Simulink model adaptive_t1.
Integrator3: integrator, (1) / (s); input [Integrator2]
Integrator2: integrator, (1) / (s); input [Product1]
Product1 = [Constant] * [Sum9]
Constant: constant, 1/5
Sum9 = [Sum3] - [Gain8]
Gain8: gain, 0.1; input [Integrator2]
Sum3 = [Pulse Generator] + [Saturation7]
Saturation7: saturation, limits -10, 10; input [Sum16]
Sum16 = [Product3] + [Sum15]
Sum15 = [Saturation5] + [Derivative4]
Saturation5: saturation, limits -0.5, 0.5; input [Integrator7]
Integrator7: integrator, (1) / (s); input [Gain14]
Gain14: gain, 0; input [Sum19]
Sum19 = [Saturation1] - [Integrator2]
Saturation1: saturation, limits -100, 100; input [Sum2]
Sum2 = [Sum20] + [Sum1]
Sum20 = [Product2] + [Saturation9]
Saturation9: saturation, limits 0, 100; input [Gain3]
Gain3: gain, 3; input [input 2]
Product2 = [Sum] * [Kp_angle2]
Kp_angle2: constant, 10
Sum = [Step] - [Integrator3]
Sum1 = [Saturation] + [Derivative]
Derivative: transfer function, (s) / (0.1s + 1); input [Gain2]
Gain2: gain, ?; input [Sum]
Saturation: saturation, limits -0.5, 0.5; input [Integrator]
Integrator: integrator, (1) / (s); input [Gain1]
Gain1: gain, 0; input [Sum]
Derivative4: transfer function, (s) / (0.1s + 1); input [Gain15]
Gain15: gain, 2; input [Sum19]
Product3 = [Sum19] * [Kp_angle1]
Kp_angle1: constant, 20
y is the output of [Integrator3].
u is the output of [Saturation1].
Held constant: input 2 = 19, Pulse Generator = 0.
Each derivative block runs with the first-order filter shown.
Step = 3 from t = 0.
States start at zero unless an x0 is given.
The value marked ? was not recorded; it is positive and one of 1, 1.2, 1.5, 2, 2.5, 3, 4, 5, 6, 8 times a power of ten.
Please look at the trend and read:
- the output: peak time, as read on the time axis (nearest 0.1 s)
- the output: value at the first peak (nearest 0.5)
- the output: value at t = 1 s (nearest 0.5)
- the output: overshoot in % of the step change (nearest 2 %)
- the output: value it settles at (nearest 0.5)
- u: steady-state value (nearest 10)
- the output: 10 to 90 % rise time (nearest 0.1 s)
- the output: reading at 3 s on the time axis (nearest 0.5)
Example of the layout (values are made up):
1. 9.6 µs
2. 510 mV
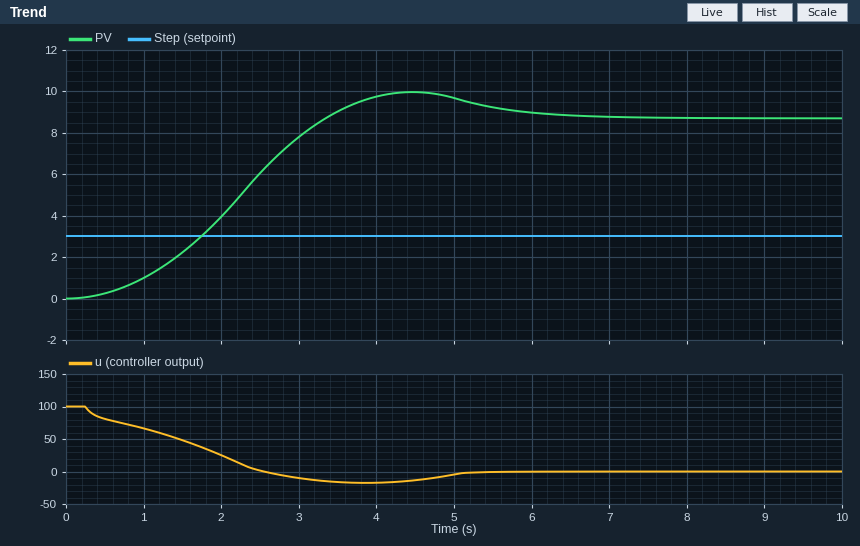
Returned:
1. 4.5 s
2. 10.0
3. 1.0
4. 14 %
5. 8.5
6. 0
7. 2.1 s
8. 8.0
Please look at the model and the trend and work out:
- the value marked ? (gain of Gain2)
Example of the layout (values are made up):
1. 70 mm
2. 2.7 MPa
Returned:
1. 6
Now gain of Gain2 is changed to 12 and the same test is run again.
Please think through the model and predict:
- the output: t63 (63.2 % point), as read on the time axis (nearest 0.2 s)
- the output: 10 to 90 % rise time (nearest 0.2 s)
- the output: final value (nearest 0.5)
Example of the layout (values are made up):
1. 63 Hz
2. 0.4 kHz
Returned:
1. 2.6 s
2. 3.4 s
3. 8.5
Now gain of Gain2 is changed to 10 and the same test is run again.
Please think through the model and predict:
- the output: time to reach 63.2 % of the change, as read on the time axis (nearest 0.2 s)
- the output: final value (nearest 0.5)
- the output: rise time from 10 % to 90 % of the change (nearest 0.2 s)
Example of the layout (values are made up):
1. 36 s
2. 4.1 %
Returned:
1. 2.4 s
2. 8.5
3. 2.8 s
